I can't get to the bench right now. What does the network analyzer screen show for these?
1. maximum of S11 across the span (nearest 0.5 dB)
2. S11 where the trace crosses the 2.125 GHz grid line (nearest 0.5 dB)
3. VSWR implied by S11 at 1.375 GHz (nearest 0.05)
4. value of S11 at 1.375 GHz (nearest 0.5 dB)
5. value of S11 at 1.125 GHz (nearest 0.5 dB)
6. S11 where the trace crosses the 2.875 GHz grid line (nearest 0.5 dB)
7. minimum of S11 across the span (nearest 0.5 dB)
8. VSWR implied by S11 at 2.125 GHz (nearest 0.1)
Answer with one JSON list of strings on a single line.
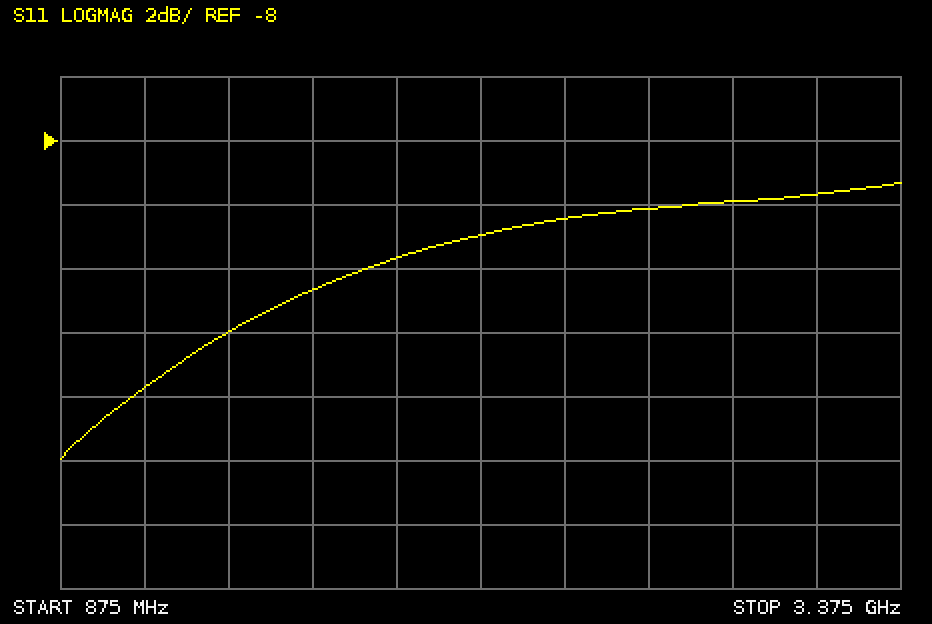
["-9.5 dB", "-11.0 dB", "1.50", "-14.0 dB", "-15.5 dB", "-10.0 dB", "-18.0 dB", "1.8"]
